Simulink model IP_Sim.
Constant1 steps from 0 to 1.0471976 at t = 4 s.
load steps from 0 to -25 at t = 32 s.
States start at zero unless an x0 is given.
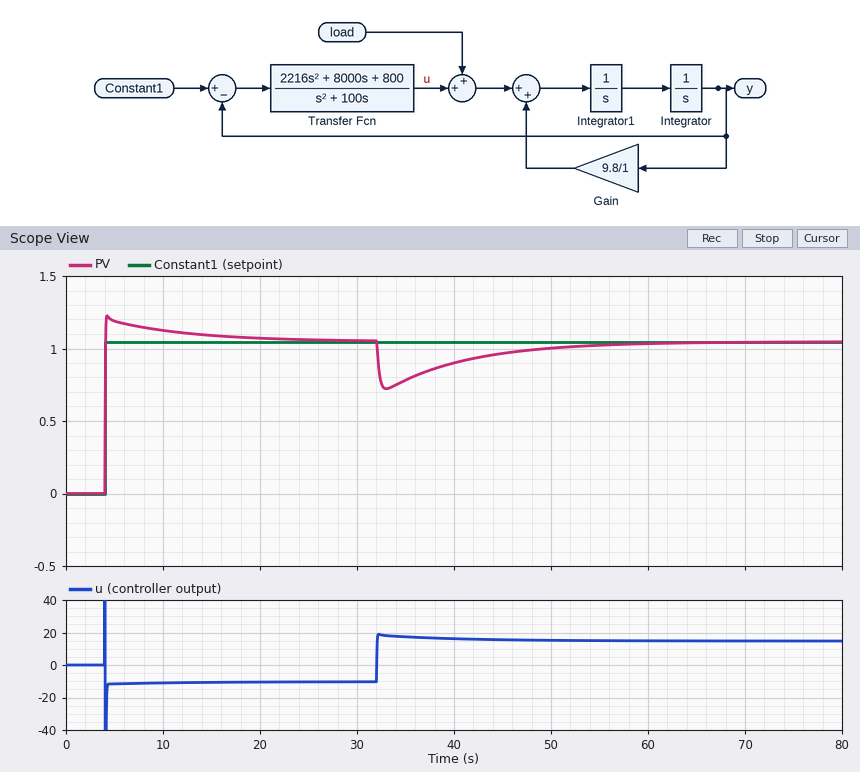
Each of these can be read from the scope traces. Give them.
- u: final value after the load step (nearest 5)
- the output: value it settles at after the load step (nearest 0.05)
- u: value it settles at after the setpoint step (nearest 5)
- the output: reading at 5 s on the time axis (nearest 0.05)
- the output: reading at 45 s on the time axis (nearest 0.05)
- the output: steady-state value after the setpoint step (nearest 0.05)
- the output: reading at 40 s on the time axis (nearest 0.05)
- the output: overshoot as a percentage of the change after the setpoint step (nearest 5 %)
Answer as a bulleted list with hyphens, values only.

- 15
- 1.05
- -10
- 1.20
- 0.95
- 1.05
- 0.90
- 15 %
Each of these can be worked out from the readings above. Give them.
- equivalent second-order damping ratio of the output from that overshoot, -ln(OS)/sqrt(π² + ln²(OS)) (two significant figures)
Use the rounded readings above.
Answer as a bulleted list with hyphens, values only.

- 0.52
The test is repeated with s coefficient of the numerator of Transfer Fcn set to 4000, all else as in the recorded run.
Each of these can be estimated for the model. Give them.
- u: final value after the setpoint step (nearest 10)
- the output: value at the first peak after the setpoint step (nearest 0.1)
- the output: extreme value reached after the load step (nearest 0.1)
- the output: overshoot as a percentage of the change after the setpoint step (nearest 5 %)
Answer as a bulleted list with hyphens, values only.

- -10
- 1.3
- 0.4
- 25 %
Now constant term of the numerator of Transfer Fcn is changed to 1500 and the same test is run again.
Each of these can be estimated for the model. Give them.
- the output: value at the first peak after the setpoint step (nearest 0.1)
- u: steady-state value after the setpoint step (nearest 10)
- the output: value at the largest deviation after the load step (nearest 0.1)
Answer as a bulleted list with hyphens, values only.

- 1.2
- -10
- 0.7
